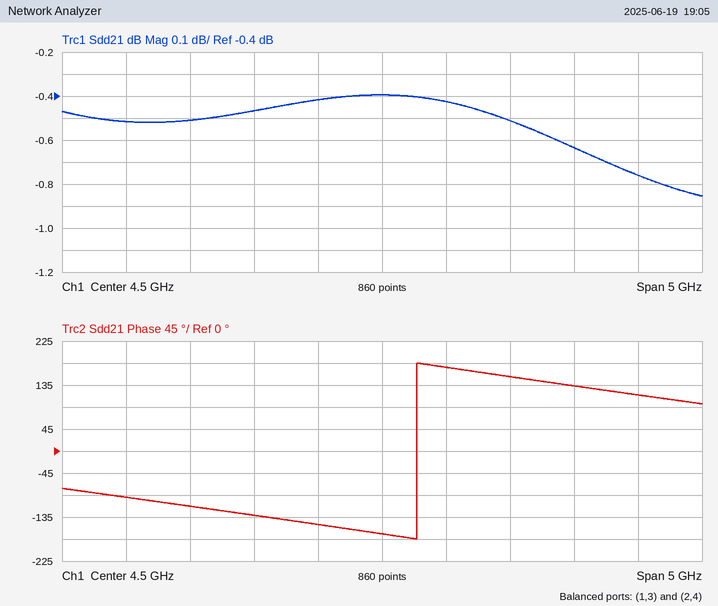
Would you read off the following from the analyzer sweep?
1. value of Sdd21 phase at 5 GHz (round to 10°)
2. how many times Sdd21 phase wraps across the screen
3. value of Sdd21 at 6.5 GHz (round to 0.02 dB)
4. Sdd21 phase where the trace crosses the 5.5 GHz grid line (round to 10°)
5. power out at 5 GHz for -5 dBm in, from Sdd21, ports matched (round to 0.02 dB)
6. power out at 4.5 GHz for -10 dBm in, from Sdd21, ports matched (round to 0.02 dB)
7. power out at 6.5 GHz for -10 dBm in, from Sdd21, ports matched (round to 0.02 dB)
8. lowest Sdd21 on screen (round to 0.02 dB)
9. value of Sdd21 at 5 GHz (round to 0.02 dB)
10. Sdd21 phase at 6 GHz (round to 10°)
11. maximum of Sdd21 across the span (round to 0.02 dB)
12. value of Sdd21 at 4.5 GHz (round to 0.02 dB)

170°
1
-0.76 dB
150°
-5.42 dBm
-10.40 dBm
-10.76 dBm
-0.86 dB
-0.42 dB
130°
-0.40 dB
-0.40 dB
